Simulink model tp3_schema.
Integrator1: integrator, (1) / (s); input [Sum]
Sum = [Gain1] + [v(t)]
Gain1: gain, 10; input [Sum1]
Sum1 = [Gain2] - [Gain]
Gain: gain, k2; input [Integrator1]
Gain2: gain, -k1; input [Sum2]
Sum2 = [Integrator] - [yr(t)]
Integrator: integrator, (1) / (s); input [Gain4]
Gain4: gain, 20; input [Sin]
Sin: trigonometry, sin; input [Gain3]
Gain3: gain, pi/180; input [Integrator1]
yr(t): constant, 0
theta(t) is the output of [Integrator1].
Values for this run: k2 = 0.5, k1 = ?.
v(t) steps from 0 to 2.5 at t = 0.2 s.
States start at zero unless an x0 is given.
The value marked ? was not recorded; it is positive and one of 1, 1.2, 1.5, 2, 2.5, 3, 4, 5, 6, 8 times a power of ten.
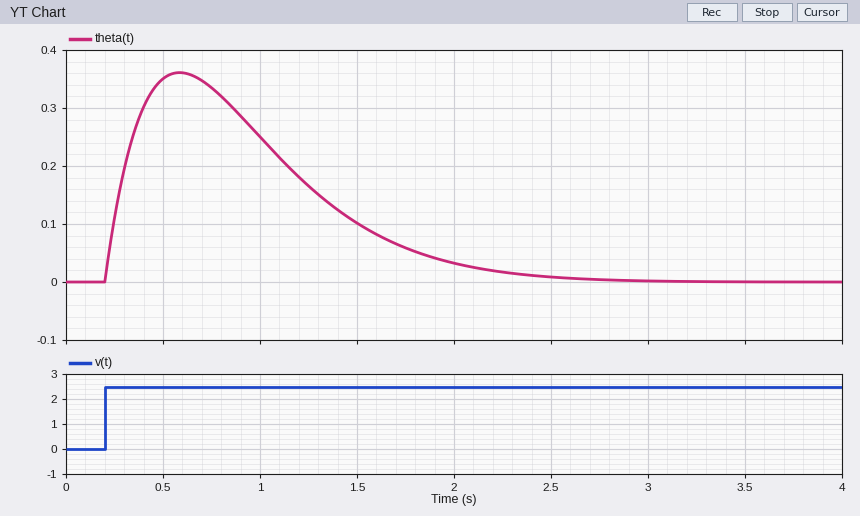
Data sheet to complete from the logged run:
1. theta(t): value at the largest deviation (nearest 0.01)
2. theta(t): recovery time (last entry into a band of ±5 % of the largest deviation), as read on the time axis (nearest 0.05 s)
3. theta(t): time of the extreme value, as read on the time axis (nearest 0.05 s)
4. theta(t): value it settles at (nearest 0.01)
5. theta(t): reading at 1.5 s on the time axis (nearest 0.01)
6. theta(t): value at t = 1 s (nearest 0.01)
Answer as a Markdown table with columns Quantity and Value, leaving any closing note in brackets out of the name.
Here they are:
| Quantity | Value |
|---|---|
| theta(t): value at the largest deviation | 0.36 |
| theta(t): recovery time (last entry into a band of ±5 % of the largest deviation), as read on the time axis | 2.25 s |
| theta(t): time of the extreme value, as read on the time axis | 0.60 s |
| theta(t): value it settles at | 0.00 |
| theta(t): reading at 1.5 s on the time axis | 0.10 |
| theta(t): value at t = 1 s | 0.25 |
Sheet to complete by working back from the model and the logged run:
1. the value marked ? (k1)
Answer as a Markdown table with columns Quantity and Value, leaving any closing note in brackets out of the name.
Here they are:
| Quantity | Value |
|---|---|
| the value marked ? | 2 |
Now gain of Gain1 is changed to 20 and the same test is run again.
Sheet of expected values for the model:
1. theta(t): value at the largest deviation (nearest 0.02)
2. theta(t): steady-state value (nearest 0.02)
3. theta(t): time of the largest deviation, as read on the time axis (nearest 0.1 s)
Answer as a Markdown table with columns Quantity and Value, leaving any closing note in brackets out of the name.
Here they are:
| Quantity | Value |
|---|---|
| theta(t): value at the largest deviation | 0.20 |
| theta(t): steady-state value | 0.00 |
| theta(t): time of the largest deviation, as read on the time axis | 0.4 s |
